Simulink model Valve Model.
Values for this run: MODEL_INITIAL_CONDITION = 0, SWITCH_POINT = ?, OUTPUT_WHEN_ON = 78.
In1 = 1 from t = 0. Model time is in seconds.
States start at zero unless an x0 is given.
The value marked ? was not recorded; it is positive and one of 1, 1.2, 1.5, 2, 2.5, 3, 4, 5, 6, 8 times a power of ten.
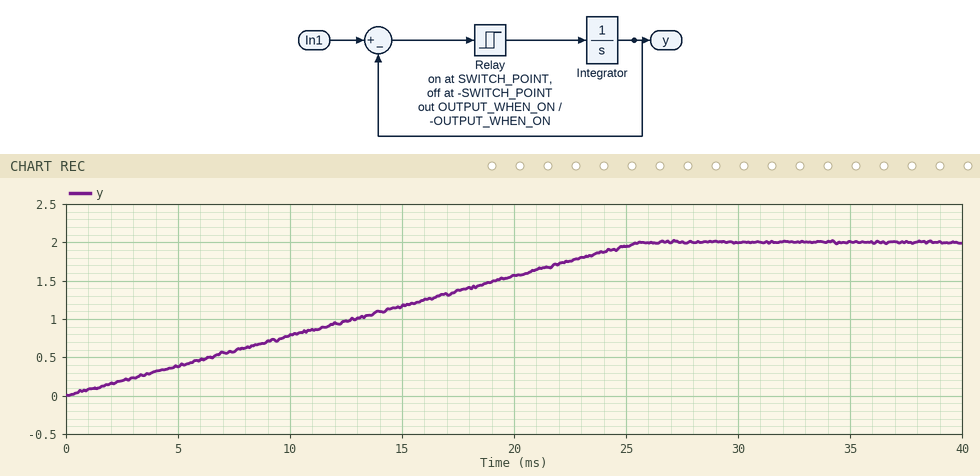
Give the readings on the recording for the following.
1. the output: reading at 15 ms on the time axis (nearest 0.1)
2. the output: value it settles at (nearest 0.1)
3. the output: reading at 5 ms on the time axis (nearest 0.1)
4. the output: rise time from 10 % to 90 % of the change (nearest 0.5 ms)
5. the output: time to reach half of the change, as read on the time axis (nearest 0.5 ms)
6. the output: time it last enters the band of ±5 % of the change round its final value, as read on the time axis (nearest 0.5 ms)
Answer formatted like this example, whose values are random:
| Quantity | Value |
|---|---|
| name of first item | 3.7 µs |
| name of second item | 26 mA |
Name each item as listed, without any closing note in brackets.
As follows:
| Quantity | Value |
|---|---|
| the output: reading at 15 ms on the time axis | 1.2 |
| the output: value it settles at | 2.0 |
| the output: reading at 5 ms on the time axis | 0.4 |
| the output: rise time from 10 % to 90 % of the change | 20.5 ms |
| the output: time to reach half of the change, as read on the time axis | 13.0 ms |
| the output: time it last enters the band of ±5 % of the change round its final value, as read on the time axis | 24.5 ms |
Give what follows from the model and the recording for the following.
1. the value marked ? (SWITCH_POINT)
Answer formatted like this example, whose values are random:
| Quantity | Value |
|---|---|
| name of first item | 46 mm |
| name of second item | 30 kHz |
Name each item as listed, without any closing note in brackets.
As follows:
| Quantity | Value |
|---|---|
| the value marked ? | 1 |
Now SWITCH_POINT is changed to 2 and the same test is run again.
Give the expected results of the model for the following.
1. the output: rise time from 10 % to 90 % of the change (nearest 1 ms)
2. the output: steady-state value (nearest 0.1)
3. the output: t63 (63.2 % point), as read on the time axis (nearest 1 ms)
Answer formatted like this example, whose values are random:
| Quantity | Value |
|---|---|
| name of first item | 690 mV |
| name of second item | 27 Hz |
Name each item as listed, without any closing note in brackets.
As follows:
| Quantity | Value |
|---|---|
| the output: rise time from 10 % to 90 % of the change | 10 ms |
| the output: steady-state value | -1.0 |
| the output: t63 (63.2 % point), as read on the time axis | 8 ms |
